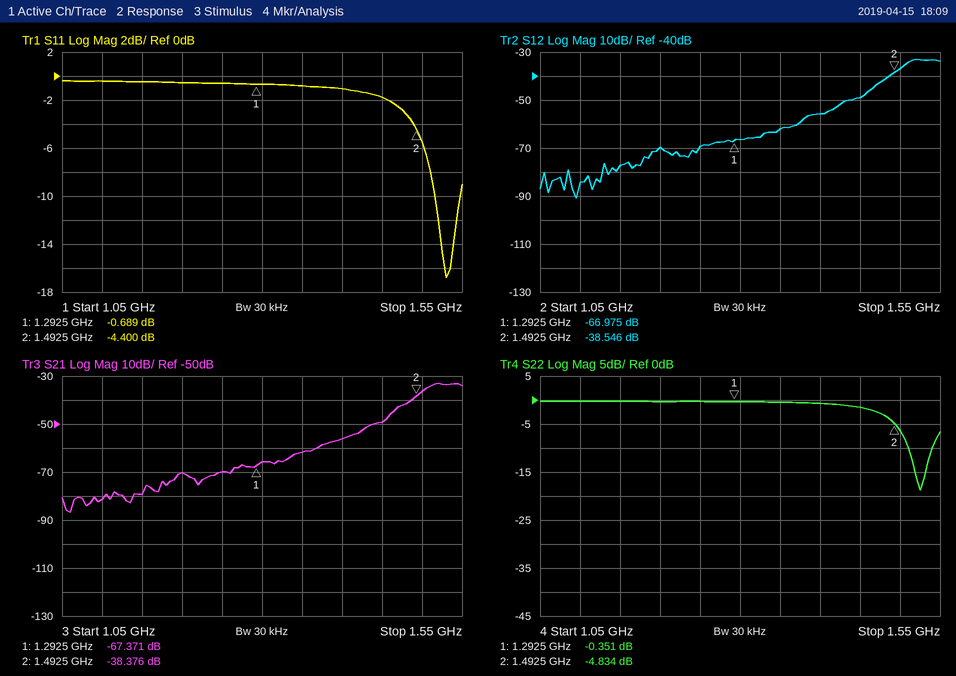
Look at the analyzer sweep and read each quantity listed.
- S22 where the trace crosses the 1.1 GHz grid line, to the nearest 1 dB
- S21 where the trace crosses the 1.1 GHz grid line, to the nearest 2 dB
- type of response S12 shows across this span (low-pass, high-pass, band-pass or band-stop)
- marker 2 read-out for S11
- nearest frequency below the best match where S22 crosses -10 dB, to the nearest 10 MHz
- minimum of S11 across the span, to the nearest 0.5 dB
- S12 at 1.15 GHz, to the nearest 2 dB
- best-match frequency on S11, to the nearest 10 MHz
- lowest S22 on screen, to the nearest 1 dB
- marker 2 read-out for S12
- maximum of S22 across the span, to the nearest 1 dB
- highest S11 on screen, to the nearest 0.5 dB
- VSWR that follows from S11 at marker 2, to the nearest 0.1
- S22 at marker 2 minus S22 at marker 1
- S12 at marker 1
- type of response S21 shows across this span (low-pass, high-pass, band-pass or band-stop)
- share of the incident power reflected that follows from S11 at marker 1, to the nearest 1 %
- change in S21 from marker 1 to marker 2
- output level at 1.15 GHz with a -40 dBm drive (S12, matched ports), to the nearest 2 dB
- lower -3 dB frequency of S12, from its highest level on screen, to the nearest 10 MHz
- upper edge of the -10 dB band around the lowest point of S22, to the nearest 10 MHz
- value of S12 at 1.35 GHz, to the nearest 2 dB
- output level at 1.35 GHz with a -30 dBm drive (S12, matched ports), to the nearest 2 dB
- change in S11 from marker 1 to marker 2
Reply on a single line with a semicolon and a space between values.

0 dB; -82 dB; high-pass; -4.400 dB; 1.51 GHz; -17.0 dB; -78 dB; 1.53 GHz; -19 dB; -38.546 dB; 0 dB; -0.5 dB; 4.0; -4.483 dB; -66.975 dB; high-pass; 85 %; 28.995 dB; -118 dBm; 1.50 GHz; 1.54 GHz; -62 dB; -92 dBm; -3.711 dB
